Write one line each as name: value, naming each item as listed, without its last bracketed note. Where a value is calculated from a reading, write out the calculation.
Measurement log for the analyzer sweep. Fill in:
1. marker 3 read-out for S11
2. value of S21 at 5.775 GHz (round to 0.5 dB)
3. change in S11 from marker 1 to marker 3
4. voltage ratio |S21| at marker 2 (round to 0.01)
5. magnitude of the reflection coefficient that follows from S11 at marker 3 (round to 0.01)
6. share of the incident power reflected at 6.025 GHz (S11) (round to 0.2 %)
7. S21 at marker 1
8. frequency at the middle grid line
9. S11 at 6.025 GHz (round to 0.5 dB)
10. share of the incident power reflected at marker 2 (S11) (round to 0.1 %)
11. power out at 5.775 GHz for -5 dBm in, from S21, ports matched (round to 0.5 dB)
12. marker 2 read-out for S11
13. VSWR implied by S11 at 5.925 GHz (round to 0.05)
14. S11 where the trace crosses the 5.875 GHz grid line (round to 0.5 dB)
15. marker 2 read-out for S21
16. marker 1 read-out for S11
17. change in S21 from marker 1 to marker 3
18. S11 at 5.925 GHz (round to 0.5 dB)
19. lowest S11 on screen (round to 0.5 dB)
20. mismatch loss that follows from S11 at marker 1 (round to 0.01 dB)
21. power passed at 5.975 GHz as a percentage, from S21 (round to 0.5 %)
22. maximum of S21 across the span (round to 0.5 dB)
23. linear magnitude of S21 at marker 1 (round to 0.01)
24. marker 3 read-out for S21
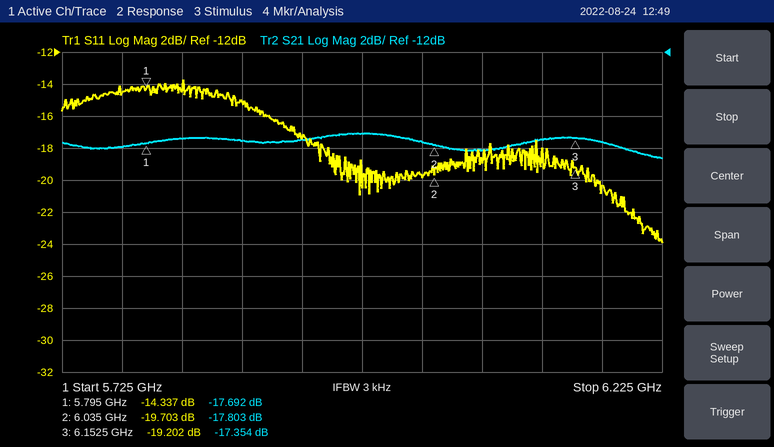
marker 3 read-out for S11: -19.202 dB
value of S21 at 5.775 GHz: -18.0 dB
change in S11 from marker 1 to marker 3: -19.202 − (-14.337) = -4.865 dB
voltage ratio |S21| at marker 2: 10^(-17.803/20) ≈ 0.13
magnitude of the reflection coefficient that follows from S11 at marker 3: 10^(-19.202/20) ≈ 0.11
share of the incident power reflected at 6.025 GHz (S11): 10^(-20/10) ≈ 1.0 %
S21 at marker 1: -17.692 dB
frequency at the middle grid line: 5.975 GHz
S11 at 6.025 GHz: -20.0 dB
share of the incident power reflected at marker 2 (S11): 10^(-19.703/10) ≈ 1.1 %
power out at 5.775 GHz for -5 dBm in, from S21, ports matched: -5 dBm + (-18.0 dB) = -23.0 dBm
marker 2 read-out for S11: -19.703 dB
VSWR implied by S11 at 5.925 GHz: |Γ| = 10^(-17.5/20) = 0.1334; VSWR = (1 + 0.1334)/(1 − 0.1334) ≈ 1.31, so 1.30 to the nearest 0.05
S11 where the trace crosses the 5.875 GHz grid line: -15.0 dB
marker 2 read-out for S21: -17.803 dB
marker 1 read-out for S11: -14.337 dB
change in S21 from marker 1 to marker 3: -17.354 − (-17.692) = 0.338 dB
S11 at 5.925 GHz: -17.5 dB
lowest S11 on screen: -24.0 dB
mismatch loss that follows from S11 at marker 1: −10 log10(1 − 10^(-14.337/10)) ≈ 0.16 dB
power passed at 5.975 GHz as a percentage, from S21: 10^(-17/10) ≈ 2.0 %
maximum of S21 across the span: -17.0 dB
linear magnitude of S21 at marker 1: 10^(-17.692/20) ≈ 0.13
marker 3 read-out for S21: -17.354 dB
